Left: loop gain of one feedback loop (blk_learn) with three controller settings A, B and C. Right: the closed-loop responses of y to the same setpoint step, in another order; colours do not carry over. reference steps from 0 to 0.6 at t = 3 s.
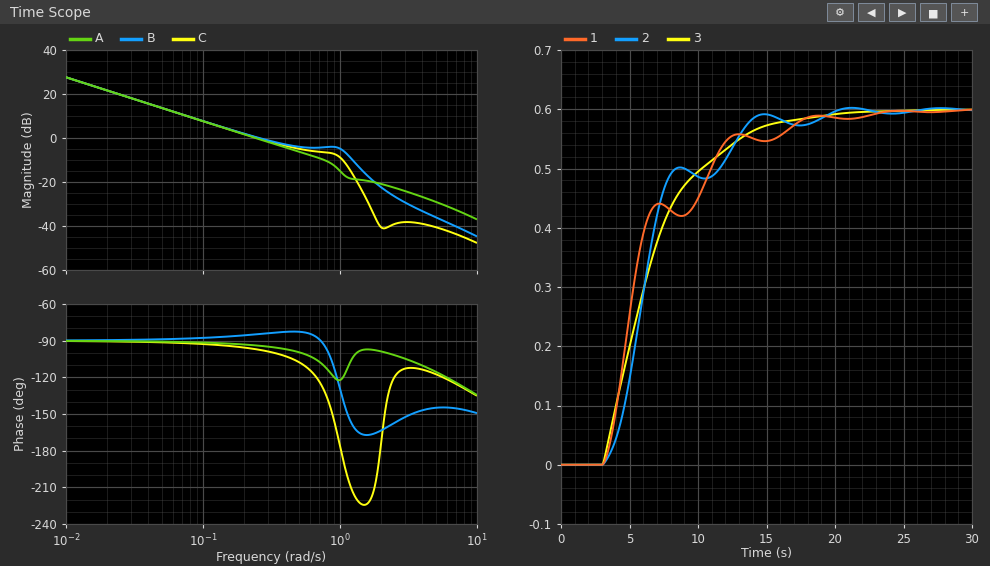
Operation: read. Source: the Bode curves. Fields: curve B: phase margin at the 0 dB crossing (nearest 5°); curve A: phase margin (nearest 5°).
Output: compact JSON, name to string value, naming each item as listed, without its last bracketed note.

{"curve B: phase margin at the 0 dB crossing": "95°", "curve A: phase margin": "85°"}
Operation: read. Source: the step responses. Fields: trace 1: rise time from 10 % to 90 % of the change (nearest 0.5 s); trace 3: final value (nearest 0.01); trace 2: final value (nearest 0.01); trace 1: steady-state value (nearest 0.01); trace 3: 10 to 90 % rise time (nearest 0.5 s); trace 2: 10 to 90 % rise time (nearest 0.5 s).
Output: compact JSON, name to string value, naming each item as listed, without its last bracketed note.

{"trace 1: rise time from 10 % to 90 % of the change": "8.0 s", "trace 3: final value": "0.60", "trace 2: final value": "0.60", "trace 1: steady-state value": "0.60", "trace 3: 10 to 90 % rise time": "9.0 s", "trace 2: 10 to 90 % rise time": "8.5 s"}
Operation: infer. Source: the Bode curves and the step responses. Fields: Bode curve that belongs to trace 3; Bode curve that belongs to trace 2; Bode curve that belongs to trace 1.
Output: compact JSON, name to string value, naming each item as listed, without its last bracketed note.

{"Bode curve that belongs to trace 3": "A", "Bode curve that belongs to trace 2": "C", "Bode curve that belongs to trace 1": "B"}
